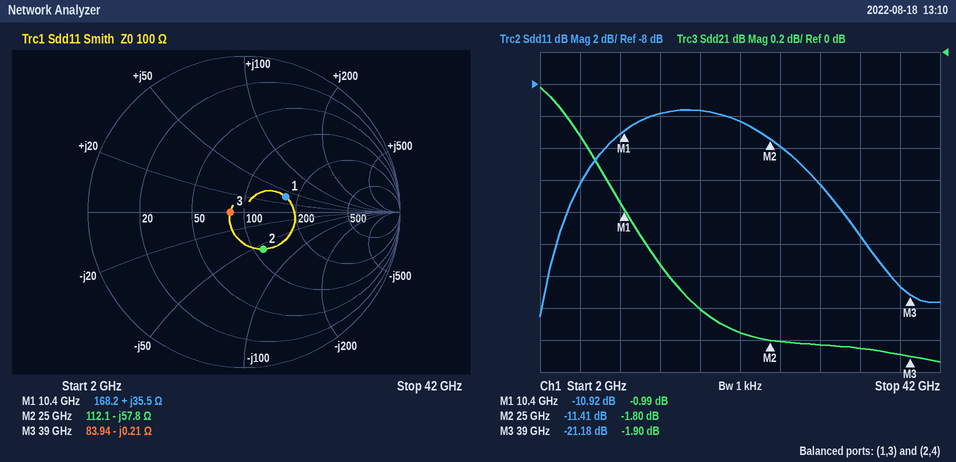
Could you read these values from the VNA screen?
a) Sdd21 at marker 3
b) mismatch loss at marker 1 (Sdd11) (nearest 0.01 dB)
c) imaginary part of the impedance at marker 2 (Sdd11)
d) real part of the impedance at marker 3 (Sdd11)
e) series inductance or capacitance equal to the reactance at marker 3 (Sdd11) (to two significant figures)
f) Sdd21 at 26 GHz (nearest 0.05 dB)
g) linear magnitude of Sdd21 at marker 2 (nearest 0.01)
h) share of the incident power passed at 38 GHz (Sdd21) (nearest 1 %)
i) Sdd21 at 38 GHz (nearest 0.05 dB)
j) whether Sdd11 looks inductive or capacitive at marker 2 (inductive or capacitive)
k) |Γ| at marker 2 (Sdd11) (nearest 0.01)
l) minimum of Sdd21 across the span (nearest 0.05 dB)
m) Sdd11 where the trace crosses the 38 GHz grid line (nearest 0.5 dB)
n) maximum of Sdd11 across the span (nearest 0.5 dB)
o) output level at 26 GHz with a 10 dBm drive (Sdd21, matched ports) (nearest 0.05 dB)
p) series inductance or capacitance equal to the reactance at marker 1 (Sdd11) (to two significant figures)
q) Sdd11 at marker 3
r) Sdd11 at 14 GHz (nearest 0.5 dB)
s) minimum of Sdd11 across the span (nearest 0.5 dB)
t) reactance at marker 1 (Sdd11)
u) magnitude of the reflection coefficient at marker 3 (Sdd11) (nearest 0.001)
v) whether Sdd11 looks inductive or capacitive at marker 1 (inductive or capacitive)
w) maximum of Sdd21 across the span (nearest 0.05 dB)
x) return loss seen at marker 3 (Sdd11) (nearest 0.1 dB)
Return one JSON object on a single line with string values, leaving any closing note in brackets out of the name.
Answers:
{"Sdd21 at marker 3": "-1.90 dB", "mismatch loss at marker 1 (Sdd11)": "0.37 dB", "imaginary part of the impedance at marker 2": "-57.8 Ω", "real part of the impedance at marker 3": "83.94 Ω", "series inductance or capacitance equal to the reactance at marker 3 (Sdd11)": "19 pF", "Sdd21 at 26 GHz": "-1.80 dB", "linear magnitude of Sdd21 at marker 2": "0.81", "share of the incident power passed at 38 GHz (Sdd21)": "65 %", "Sdd21 at 38 GHz": "-1.90 dB", "whether Sdd11 looks inductive or capacitive at marker 2": "capacitive", "|Γ| at marker 2 (Sdd11)": "0.27", "minimum of Sdd21 across the span": "-1.95 dB", "Sdd11 where the trace crosses the 38 GHz grid line": "-20.5 dB", "maximum of Sdd11 across the span": "-9.5 dB", "output level at 26 GHz with a 10 dBm drive (Sdd21, matched ports)": "8.20 dBm", "series inductance or capacitance equal to the reactance at marker 1 (Sdd11)": "540 pH", "Sdd11 at marker 3": "-21.18 dB", "Sdd11 at 14 GHz": "-10.0 dB", "minimum of Sdd11 across the span": "-22.5 dB", "reactance at marker 1": "+35.5 Ω", "magnitude of the reflection coefficient at marker 3 (Sdd11)": "0.087", "whether Sdd11 looks inductive or capacitive at marker 1": "inductive", "maximum of Sdd21 across the span": "-0.20 dB", "return loss seen at marker 3 (Sdd11)": "21.2 dB"}
